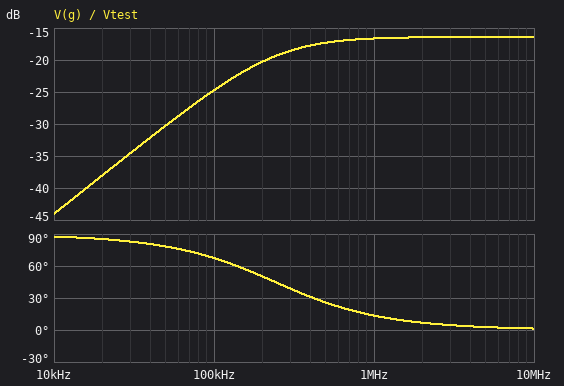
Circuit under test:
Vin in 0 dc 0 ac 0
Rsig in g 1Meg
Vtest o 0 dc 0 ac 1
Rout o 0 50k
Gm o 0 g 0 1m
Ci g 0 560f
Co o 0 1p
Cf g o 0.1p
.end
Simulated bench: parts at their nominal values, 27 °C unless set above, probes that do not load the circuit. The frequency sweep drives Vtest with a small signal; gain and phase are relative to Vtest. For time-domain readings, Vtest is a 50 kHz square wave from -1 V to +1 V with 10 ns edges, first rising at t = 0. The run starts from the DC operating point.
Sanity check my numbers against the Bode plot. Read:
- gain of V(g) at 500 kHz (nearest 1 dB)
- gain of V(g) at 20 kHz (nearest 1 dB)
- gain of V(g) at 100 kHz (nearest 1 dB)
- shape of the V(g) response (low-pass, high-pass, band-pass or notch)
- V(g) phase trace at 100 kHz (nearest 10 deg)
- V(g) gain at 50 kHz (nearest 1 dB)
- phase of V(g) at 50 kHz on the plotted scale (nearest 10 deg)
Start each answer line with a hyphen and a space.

- -17 dB
- -38 dB
- -25 dB
- high-pass
- 70 deg
- -30 dB
- 80 deg
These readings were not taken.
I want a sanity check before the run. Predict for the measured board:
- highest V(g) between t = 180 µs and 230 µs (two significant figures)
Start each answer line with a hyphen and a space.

- 300 mV
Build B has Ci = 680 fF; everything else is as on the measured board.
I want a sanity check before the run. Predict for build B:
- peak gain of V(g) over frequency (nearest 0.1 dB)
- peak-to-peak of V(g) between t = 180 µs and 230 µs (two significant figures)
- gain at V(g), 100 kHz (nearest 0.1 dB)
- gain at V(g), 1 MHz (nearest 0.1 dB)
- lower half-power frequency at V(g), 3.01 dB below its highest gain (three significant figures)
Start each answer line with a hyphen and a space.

- -17.8 dB
- 510 mV
- -25.0 dB
- -18.0 dB
- 204 kHz
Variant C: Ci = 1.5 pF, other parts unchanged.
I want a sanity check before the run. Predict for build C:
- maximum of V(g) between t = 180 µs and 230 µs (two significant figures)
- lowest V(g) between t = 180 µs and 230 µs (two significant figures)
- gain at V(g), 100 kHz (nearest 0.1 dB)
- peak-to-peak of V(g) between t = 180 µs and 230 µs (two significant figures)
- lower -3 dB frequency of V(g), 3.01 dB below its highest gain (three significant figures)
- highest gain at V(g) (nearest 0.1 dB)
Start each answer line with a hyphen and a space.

- 120 mV
- -120 mV
- -27.1 dB
- 250 mV
- 99.5 kHz
- -24.1 dB
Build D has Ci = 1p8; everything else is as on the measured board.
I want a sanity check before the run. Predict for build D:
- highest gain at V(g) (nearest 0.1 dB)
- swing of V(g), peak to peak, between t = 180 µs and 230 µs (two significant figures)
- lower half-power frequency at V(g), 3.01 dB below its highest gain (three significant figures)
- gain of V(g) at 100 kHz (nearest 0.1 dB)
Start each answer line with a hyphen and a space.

- -25.6 dB
- 210 mV
- 83.8 kHz
- -27.9 dB
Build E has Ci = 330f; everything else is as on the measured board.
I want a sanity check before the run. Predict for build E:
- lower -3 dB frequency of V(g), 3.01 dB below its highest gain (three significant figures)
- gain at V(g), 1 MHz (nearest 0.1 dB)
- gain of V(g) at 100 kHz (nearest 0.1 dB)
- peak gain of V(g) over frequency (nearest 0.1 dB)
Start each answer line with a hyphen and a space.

- 370 kHz
- -13.2 dB
- -24.3 dB
- -12.7 dB
